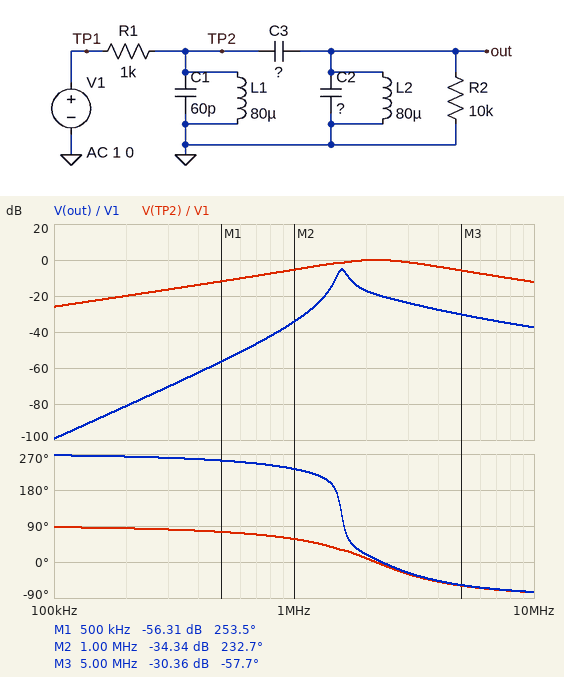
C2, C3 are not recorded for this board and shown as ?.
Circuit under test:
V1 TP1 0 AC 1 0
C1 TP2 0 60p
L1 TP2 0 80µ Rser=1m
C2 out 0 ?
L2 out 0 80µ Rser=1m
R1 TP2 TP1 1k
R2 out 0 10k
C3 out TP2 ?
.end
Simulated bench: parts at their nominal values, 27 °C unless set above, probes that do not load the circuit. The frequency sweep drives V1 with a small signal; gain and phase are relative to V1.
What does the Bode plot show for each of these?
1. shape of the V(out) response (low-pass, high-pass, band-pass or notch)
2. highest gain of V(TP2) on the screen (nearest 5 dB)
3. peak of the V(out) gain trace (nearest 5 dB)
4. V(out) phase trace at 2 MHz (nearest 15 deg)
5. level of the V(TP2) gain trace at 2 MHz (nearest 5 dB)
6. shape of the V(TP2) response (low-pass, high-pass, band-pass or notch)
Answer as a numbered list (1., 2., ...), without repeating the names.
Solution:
1. band-pass
2. 0 dB
3. -5 dB
4. 15 deg
5. 0 dB
6. band-pass
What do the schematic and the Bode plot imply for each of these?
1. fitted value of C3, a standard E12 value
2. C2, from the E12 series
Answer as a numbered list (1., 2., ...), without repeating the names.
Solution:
1. 6.8 pF
2. 120 pF
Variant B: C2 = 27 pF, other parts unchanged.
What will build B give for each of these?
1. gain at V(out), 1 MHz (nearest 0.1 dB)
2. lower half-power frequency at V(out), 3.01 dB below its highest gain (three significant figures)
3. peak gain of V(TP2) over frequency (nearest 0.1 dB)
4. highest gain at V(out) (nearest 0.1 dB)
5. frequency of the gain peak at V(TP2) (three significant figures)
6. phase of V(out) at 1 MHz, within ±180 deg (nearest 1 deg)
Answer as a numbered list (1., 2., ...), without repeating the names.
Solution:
1. -37.8 dB
2. 2.83 MHz
3. 0 dB
4. -0.1 dB
5. 2.14 MHz
6. -126 deg
